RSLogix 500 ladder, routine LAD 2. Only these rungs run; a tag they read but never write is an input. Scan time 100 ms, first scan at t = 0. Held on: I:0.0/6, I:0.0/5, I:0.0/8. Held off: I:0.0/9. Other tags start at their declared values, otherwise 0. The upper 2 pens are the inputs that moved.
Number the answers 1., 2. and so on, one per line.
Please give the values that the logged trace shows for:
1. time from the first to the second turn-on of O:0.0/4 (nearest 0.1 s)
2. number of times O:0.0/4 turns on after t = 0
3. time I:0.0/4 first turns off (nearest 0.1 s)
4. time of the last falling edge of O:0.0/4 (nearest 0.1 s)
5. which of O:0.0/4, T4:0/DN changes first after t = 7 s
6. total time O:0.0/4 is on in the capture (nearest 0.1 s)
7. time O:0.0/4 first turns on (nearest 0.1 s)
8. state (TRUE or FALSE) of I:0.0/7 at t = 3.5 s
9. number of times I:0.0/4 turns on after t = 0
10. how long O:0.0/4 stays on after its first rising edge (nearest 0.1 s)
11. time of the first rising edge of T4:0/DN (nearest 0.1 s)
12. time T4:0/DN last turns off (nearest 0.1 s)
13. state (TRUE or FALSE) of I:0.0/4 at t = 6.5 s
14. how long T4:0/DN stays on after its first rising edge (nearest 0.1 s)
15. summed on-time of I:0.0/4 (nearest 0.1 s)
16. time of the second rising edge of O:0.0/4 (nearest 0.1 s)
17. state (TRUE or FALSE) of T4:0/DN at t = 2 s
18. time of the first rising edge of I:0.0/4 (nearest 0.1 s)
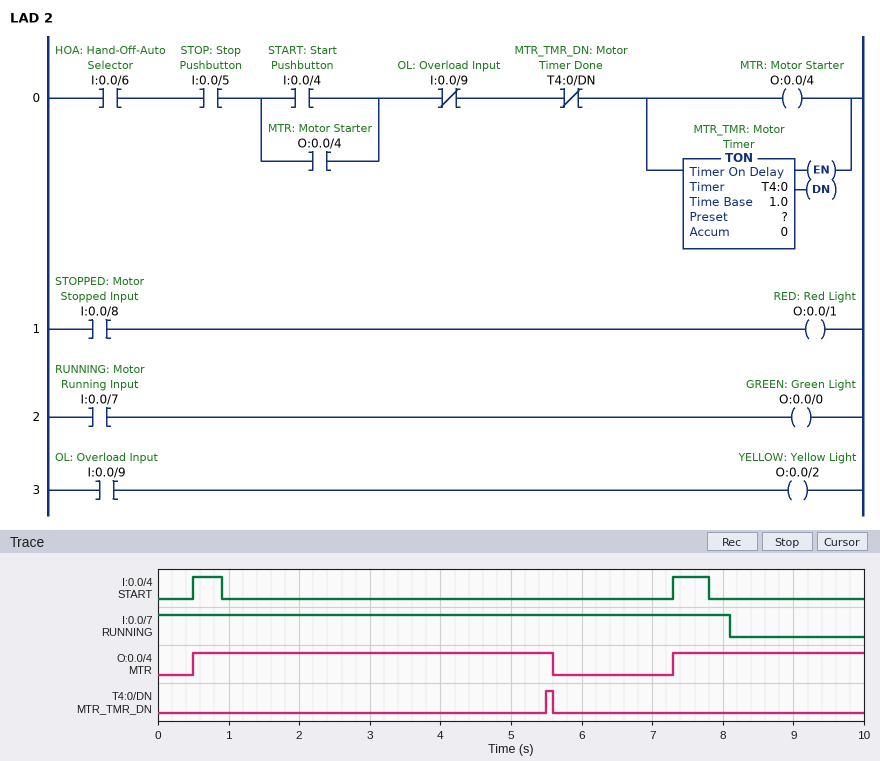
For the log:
1. 6.8 s
2. 2
3. 0.9 s
4. 5.6 s
5. O:0.0/4
6. 7.8 s
7. 0.5 s
8. TRUE
9. 2
10. 5.1 s
11. 5.5 s
12. 5.6 s
13. FALSE
14. 0.1 s
15. 0.9 s
16. 7.3 s
17. FALSE
18. 0.5 s
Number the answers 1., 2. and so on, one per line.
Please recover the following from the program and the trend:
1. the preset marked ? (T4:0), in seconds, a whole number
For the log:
1. 5 s
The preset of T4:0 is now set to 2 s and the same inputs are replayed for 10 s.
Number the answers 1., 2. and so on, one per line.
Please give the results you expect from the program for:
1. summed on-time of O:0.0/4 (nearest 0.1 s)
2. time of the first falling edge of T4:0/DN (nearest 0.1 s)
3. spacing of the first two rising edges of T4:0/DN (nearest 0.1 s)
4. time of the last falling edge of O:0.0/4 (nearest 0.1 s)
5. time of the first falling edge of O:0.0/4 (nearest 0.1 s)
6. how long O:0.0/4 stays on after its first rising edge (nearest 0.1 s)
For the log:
1. 4.2 s
2. 2.6 s
3. 6.8 s
4. 9.4 s
5. 2.6 s
6. 2.1 s
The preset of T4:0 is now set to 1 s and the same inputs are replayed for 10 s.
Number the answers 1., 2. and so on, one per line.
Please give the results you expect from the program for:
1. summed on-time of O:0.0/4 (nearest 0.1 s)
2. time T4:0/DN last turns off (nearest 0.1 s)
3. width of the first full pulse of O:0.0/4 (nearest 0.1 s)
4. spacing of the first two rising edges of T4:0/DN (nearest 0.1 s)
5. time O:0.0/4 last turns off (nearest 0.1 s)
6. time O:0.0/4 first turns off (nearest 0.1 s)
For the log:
1. 2.2 s
2. 8.4 s
3. 1.1 s
4. 6.8 s
5. 8.4 s
6. 1.6 s
